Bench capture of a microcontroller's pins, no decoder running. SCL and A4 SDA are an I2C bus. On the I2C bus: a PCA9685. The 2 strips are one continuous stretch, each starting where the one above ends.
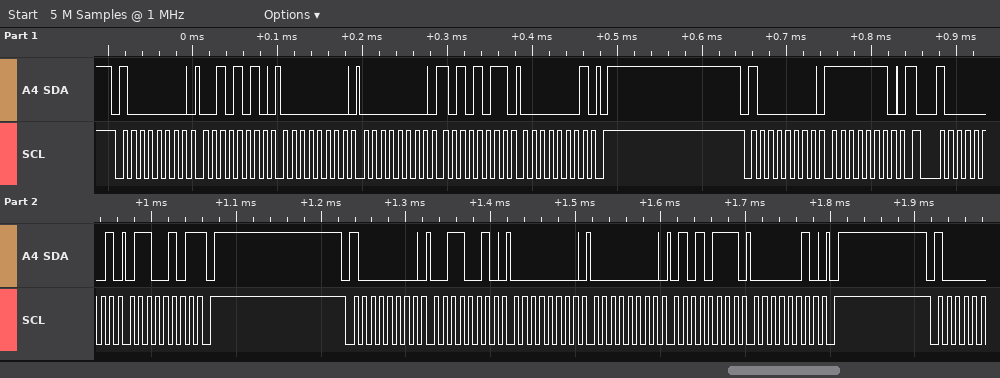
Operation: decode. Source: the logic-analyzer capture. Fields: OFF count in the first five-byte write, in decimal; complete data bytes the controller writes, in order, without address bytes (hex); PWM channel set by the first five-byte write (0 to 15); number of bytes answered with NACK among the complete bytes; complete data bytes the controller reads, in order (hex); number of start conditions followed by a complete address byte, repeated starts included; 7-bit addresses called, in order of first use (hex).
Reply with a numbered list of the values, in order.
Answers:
1. 427
2. 2A 00 00 AB 01 FE 32 00 00 57 02
3. 9
4. 1
5. 65
6. 4
7. 0x40
